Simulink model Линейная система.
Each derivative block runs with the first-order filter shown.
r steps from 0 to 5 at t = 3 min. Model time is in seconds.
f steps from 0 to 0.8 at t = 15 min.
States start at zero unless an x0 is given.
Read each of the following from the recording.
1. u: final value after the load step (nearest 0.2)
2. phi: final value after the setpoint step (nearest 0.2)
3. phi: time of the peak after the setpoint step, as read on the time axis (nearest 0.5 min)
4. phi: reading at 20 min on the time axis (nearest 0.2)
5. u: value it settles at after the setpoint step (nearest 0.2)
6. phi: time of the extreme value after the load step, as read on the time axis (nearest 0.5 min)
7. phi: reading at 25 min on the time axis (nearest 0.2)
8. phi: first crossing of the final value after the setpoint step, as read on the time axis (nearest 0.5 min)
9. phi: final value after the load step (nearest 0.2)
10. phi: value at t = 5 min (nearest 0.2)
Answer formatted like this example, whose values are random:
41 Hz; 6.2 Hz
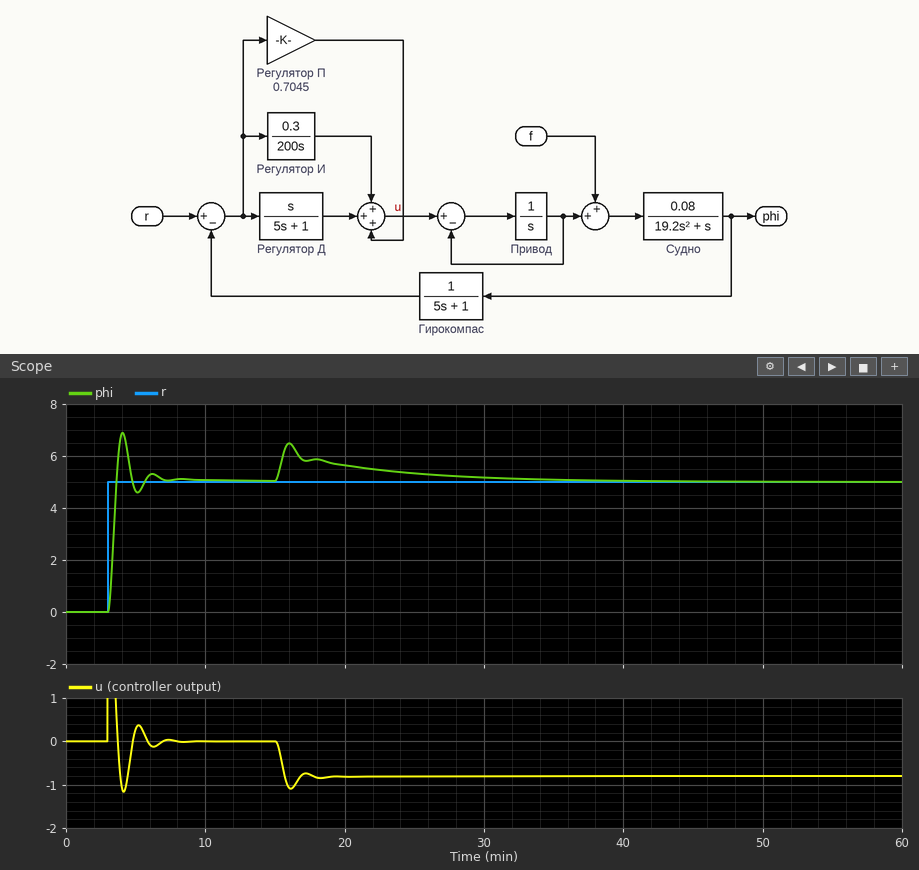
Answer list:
-0.8; 5.0; 4.0 min; 5.6; 0.0; 16.0 min; 5.4; 3.5 min; 5.0; 4.6
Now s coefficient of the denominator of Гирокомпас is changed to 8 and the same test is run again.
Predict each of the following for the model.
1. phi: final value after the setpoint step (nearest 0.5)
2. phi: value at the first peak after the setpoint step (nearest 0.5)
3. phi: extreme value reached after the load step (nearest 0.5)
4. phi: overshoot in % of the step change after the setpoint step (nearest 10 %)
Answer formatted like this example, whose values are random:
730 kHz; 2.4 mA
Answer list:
5.0; 7.5; 6.5; 50 %
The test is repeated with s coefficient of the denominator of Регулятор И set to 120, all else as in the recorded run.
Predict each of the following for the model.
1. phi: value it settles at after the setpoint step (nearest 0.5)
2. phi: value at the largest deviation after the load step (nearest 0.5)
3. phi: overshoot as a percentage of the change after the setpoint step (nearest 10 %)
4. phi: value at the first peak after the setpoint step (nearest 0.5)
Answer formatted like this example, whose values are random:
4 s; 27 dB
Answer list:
5.0; 6.5; 40 %; 7.0
